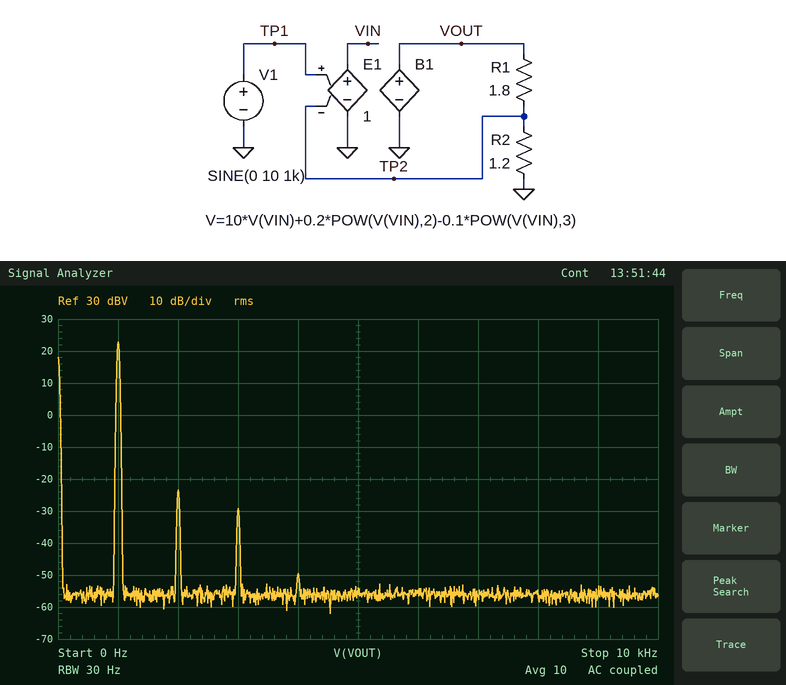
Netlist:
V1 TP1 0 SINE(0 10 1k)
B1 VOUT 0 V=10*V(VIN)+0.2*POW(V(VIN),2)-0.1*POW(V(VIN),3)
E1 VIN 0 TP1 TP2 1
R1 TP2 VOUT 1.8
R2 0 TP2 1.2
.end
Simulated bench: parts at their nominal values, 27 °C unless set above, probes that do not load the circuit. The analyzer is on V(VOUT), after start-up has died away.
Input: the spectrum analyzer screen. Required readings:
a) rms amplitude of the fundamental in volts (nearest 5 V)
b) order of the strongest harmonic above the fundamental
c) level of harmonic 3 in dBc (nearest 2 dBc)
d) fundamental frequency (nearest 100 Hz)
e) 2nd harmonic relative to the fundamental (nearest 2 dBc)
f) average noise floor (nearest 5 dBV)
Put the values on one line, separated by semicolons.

15 V; 2; -52 dBc; 1.0 kHz; -46 dBc; -55 dBV
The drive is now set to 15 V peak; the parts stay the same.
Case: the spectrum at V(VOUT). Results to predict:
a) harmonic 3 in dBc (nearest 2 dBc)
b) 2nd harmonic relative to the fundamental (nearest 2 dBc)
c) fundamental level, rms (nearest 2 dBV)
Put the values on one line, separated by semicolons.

-42 dBc; -40 dBc; 26 dBV
